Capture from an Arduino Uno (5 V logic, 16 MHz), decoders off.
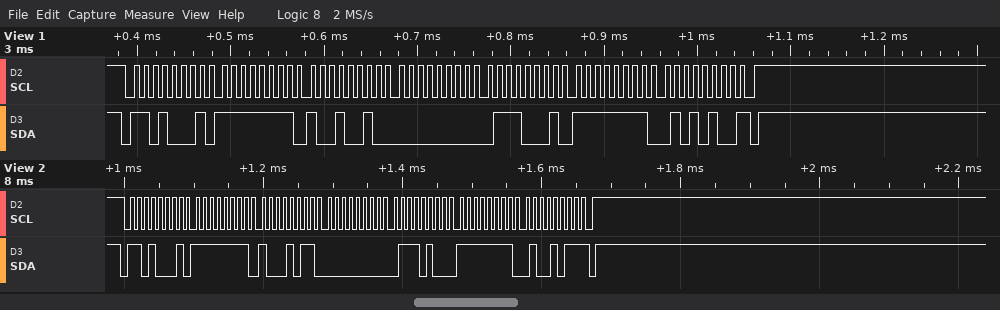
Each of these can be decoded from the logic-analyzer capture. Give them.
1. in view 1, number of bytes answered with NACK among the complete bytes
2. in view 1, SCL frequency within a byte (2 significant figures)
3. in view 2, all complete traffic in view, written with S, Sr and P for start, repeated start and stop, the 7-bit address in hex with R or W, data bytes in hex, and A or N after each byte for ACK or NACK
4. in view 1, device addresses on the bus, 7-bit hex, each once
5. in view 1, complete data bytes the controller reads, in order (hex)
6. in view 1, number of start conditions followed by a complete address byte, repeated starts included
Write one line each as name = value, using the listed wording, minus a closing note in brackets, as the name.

in view 1, number of bytes answered with NACK among the complete bytes = 1
in view 1, SCL frequency within a byte = 100 kHz
in view 2, all complete traffic in view, written with S, Sr and P for start, repeated start and stop, the 7-bit address in hex with R or W, data bytes in hex, and A or N after each byte for ACK or NACK = S 68R A FF A 8B A 00 A 74 A FF A 4B N P
in view 1, device addresses on the bus, 7-bit hex, each once = 0x68
in view 1, complete data bytes the controller reads, in order = FF 92 00 71 FF 54
in view 1, number of start conditions followed by a complete address byte, repeated starts included = 1
